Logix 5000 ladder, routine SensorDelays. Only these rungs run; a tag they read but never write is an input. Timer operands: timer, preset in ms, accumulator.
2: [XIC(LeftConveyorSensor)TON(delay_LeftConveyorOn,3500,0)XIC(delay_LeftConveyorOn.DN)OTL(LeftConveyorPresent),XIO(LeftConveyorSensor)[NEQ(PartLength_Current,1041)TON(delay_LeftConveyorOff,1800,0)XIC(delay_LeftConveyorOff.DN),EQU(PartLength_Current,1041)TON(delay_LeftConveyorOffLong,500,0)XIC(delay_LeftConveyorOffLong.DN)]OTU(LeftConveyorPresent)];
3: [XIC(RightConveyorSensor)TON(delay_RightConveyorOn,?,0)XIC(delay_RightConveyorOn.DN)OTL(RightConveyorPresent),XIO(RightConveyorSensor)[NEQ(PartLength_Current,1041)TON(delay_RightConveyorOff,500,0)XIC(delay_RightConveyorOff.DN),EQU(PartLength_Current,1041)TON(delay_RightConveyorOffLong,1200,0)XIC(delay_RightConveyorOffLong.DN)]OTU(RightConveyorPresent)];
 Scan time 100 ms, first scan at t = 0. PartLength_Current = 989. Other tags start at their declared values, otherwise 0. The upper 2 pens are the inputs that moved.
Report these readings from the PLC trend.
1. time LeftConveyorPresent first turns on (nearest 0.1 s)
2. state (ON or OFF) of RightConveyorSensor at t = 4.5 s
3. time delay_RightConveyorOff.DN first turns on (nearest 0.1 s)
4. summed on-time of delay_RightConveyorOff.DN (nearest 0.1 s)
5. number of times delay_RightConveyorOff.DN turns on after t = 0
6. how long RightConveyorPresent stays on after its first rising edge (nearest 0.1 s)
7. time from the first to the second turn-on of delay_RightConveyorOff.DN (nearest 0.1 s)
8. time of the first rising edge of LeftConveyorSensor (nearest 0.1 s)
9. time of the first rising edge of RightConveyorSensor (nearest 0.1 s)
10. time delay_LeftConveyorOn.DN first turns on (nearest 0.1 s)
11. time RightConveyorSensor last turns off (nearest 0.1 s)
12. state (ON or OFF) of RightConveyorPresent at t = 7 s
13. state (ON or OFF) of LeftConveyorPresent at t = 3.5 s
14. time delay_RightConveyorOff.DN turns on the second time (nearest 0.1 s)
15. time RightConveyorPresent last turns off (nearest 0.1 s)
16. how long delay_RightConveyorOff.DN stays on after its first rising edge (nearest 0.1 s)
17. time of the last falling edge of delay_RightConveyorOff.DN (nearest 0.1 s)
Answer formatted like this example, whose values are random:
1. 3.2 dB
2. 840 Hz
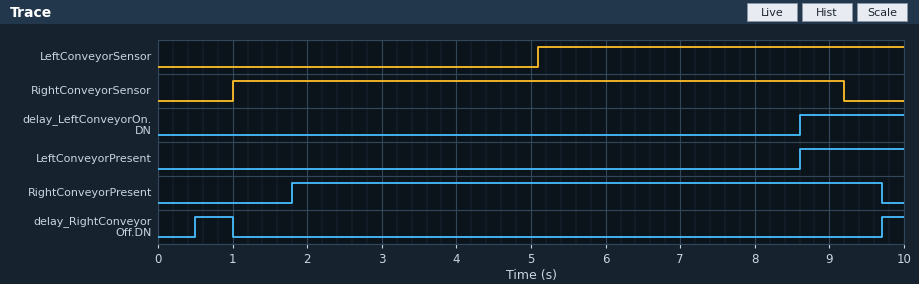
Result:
1. 8.6 s
2. ON
3. 0.5 s
4. 0.8 s
5. 2
6. 7.9 s
7. 9.2 s
8. 5.1 s
9. 1.0 s
10. 8.6 s
11. 9.2 s
12. ON
13. OFF
14. 9.7 s
15. 9.7 s
16. 0.5 s
17. 1.0 s
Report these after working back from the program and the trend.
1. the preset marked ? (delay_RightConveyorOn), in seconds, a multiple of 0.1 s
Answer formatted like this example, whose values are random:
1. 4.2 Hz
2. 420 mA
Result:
1. 0.8 s
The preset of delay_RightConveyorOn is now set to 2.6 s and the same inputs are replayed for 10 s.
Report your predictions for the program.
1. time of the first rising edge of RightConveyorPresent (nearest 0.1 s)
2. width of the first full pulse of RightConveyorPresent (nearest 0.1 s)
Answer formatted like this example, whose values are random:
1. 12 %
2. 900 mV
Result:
1. 3.6 s
2. 6.1 s
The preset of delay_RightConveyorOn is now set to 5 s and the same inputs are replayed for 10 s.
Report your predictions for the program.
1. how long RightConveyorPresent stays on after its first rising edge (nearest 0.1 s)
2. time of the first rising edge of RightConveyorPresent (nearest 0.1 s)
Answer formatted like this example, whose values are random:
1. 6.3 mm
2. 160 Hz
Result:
1. 3.7 s
2. 6.0 s
